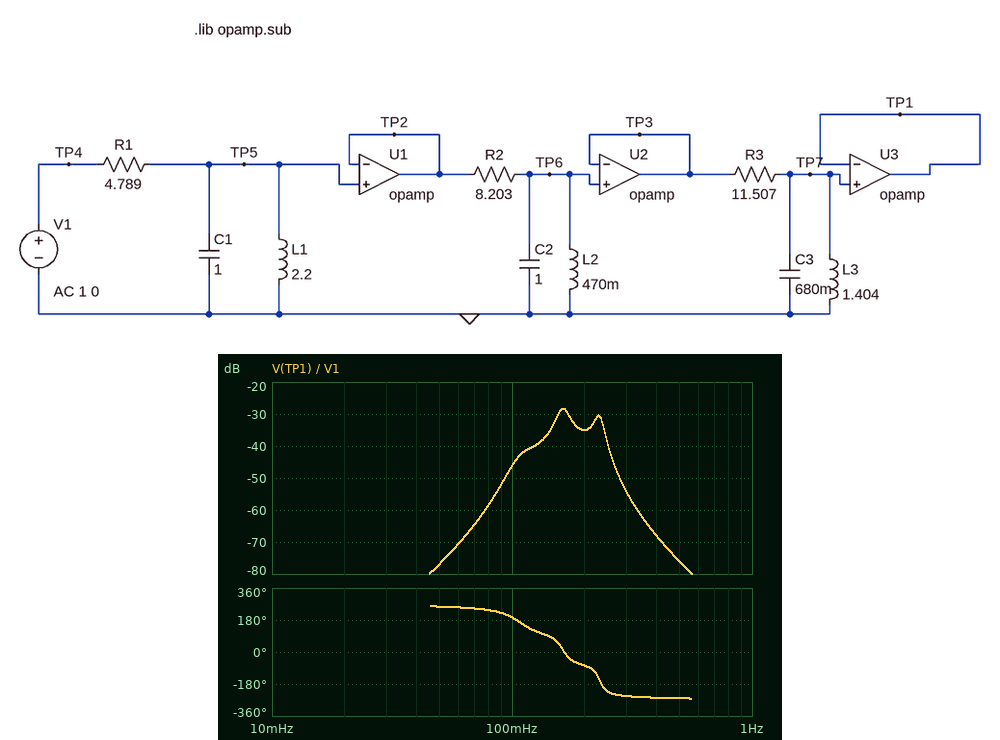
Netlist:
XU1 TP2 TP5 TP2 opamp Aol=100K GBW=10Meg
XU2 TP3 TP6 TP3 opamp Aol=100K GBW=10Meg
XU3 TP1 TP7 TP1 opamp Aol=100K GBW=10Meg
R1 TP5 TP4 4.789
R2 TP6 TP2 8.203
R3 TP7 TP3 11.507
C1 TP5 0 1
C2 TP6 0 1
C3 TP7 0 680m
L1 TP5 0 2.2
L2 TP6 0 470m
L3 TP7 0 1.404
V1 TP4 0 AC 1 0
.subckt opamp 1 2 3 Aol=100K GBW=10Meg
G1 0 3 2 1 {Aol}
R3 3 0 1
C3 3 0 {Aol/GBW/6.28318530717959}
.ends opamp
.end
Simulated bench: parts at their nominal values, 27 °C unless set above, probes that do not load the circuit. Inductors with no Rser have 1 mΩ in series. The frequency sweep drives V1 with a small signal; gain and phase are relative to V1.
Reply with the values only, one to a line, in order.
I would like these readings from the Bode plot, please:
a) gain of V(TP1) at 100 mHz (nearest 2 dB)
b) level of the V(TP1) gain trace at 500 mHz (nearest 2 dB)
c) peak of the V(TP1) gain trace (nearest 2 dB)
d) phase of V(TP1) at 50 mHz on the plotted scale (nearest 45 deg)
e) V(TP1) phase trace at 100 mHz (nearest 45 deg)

-46 dB
-76 dB
-28 dB
270 deg
180 deg
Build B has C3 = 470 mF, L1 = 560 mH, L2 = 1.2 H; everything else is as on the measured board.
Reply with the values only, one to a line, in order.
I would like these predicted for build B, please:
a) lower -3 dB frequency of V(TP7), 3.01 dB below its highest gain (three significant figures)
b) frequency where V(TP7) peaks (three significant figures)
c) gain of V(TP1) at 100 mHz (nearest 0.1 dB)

186 mHz
200 mHz
-55.6 dB
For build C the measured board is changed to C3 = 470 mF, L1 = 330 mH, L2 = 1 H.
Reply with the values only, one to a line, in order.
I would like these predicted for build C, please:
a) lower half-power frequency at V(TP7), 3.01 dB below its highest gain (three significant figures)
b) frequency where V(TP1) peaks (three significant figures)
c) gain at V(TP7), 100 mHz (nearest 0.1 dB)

158 mHz
194 mHz
-63.8 dB
